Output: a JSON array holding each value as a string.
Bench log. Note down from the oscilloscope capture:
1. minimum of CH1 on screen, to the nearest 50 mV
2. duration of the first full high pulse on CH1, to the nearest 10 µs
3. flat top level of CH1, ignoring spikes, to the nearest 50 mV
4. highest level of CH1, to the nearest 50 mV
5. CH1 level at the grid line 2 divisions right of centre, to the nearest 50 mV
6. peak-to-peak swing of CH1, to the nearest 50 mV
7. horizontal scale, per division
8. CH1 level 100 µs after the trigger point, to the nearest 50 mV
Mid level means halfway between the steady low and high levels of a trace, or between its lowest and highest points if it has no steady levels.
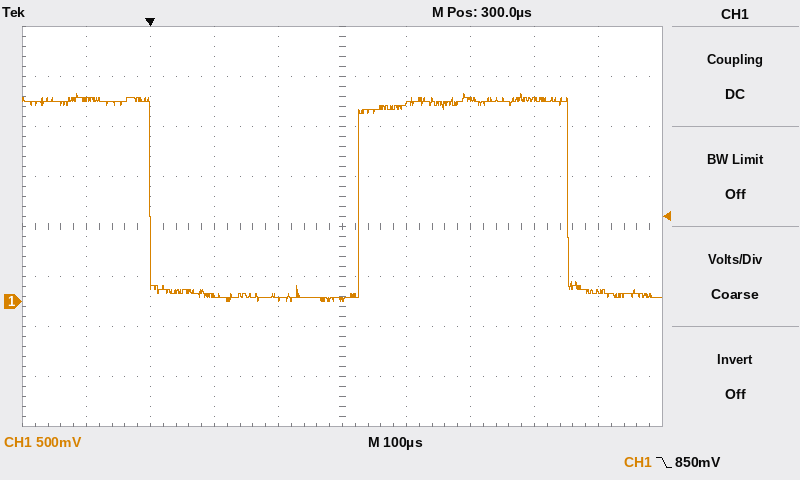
["0 mV", "330 µs", "2.00 V", "2.10 V", "2.00 V", "2.10 V", "100 µs", "50 mV"]
